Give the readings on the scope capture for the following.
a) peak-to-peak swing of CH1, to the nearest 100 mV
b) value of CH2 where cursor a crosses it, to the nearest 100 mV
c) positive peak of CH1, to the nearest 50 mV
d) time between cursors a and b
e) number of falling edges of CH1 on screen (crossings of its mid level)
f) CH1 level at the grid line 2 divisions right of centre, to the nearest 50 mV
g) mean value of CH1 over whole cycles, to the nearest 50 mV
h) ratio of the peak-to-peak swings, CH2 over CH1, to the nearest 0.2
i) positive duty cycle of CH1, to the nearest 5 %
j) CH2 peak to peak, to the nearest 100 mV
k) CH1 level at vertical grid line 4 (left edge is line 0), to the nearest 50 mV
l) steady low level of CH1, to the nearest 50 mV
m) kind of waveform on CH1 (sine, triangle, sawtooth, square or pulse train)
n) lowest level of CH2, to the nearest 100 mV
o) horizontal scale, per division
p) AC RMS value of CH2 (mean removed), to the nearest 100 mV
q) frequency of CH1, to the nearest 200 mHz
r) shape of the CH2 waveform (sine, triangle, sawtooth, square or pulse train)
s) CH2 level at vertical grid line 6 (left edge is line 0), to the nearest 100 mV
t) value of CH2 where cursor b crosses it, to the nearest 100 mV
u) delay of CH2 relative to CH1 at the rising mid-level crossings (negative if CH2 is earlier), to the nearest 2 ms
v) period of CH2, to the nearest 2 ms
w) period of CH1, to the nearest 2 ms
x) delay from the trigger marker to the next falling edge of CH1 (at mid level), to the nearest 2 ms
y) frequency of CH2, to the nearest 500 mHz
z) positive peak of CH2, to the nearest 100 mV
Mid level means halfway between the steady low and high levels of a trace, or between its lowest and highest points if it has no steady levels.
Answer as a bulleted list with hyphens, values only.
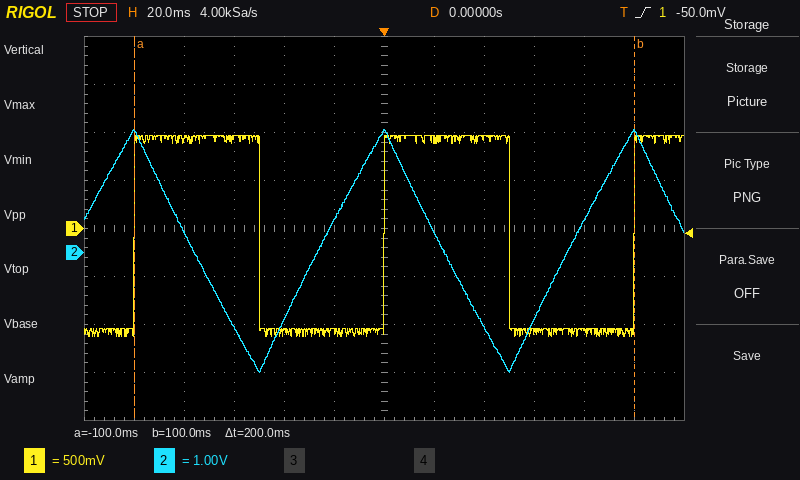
- 2.10 V
- 2.5 V
- 950 mV
- 200 ms
- 2
- 950 mV
- -50 mV
- 2.4
- 50 %
- 5.1 V
- -1.10 V
- -1.05 V
- square
- -2.5 V
- 20 ms
- 1.5 V
- 10.0 Hz
- triangle
- 2.5 V
- 2.5 V
- -26 ms
- 100 ms
- 100 ms
- 50 ms
- 10.0 Hz
- 2.6 V
